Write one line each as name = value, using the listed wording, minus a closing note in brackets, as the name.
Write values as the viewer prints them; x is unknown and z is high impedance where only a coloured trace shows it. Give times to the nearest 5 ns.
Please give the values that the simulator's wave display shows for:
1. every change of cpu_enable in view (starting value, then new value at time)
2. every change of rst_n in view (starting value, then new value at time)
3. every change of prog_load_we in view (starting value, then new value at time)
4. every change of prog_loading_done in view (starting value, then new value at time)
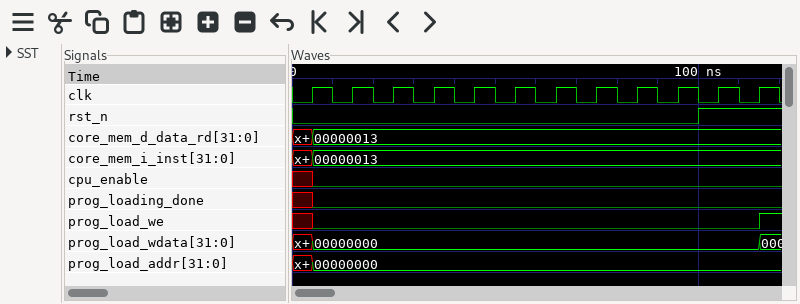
every change of cpu_enable in view = x, 0 at 5 ns
every change of rst_n in view = 0, 1 at 100 ns
every change of prog_load_we in view = x, 0 at 5 ns, 1 at 115 ns
every change of prog_loading_done in view = x, 0 at 5 ns
